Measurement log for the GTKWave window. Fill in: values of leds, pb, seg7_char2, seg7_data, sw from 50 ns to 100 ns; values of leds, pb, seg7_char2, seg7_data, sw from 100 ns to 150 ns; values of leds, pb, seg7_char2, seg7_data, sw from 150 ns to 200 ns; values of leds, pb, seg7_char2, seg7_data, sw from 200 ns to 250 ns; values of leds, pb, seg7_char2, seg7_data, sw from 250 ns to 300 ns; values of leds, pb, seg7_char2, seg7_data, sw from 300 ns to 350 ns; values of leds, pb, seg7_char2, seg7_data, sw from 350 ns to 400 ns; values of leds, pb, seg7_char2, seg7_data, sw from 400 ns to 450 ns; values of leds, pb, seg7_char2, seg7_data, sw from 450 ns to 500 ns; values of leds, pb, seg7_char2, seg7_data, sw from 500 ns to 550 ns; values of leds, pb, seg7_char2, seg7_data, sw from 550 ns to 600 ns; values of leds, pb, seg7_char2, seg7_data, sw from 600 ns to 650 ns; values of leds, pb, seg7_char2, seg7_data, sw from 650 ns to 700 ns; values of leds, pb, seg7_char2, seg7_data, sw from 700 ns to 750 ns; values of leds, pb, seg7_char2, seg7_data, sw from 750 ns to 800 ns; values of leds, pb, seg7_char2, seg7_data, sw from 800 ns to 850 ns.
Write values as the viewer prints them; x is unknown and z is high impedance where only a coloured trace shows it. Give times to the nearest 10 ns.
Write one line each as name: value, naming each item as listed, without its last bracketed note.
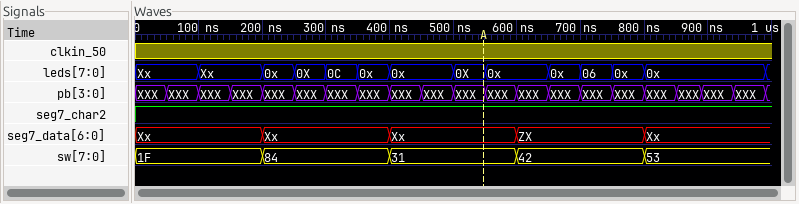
values of leds, pb, seg7_char2, seg7_data, sw from 50 ns to 100 ns: leds=Xx, pb=XXX, seg7_char2=1, seg7_data=Xx, sw=1F
values of leds, pb, seg7_char2, seg7_data, sw from 100 ns to 150 ns: leds=Xx, pb=XXX, seg7_char2=1, seg7_data=Xx, sw=1F
values of leds, pb, seg7_char2, seg7_data, sw from 150 ns to 200 ns: leds=Xx, pb=XXX, seg7_char2=1, seg7_data=Xx, sw=1F
values of leds, pb, seg7_char2, seg7_data, sw from 200 ns to 250 ns: leds=0x, pb=XXX, seg7_char2=1, seg7_data=Xx, sw=84
values of leds, pb, seg7_char2, seg7_data, sw from 250 ns to 300 ns: leds=0X, pb=XXX, seg7_char2=1, seg7_data=Xx, sw=84
values of leds, pb, seg7_char2, seg7_data, sw from 300 ns to 350 ns: leds=0C, pb=XXX, seg7_char2=1, seg7_data=Xx, sw=84
values of leds, pb, seg7_char2, seg7_data, sw from 350 ns to 400 ns: leds=0x, pb=XXX, seg7_char2=1, seg7_data=Xx, sw=84
values of leds, pb, seg7_char2, seg7_data, sw from 400 ns to 450 ns: leds=0x, pb=XXX, seg7_char2=1, seg7_data=Xx, sw=31
values of leds, pb, seg7_char2, seg7_data, sw from 450 ns to 500 ns: leds=0x, pb=XXX, seg7_char2=1, seg7_data=Xx, sw=31
values of leds, pb, seg7_char2, seg7_data, sw from 500 ns to 550 ns: leds=0X, pb=XXX, seg7_char2=1, seg7_data=Xx, sw=31
values of leds, pb, seg7_char2, seg7_data, sw from 550 ns to 600 ns: leds=0x, pb=XXX, seg7_char2=1, seg7_data=Xx, sw=31
values of leds, pb, seg7_char2, seg7_data, sw from 600 ns to 650 ns: leds=0x, pb=XXX, seg7_char2=1, seg7_data=ZX, sw=42
values of leds, pb, seg7_char2, seg7_data, sw from 650 ns to 700 ns: leds=0x, pb=XXX, seg7_char2=1, seg7_data=ZX, sw=42
values of leds, pb, seg7_char2, seg7_data, sw from 700 ns to 750 ns: leds=06, pb=XXX, seg7_char2=1, seg7_data=ZX, sw=42
values of leds, pb, seg7_char2, seg7_data, sw from 750 ns to 800 ns: leds=0x, pb=XXX, seg7_char2=1, seg7_data=ZX, sw=42
values of leds, pb, seg7_char2, seg7_data, sw from 800 ns to 850 ns: leds=0x, pb=XXX, seg7_char2=1, seg7_data=Xx, sw=53
